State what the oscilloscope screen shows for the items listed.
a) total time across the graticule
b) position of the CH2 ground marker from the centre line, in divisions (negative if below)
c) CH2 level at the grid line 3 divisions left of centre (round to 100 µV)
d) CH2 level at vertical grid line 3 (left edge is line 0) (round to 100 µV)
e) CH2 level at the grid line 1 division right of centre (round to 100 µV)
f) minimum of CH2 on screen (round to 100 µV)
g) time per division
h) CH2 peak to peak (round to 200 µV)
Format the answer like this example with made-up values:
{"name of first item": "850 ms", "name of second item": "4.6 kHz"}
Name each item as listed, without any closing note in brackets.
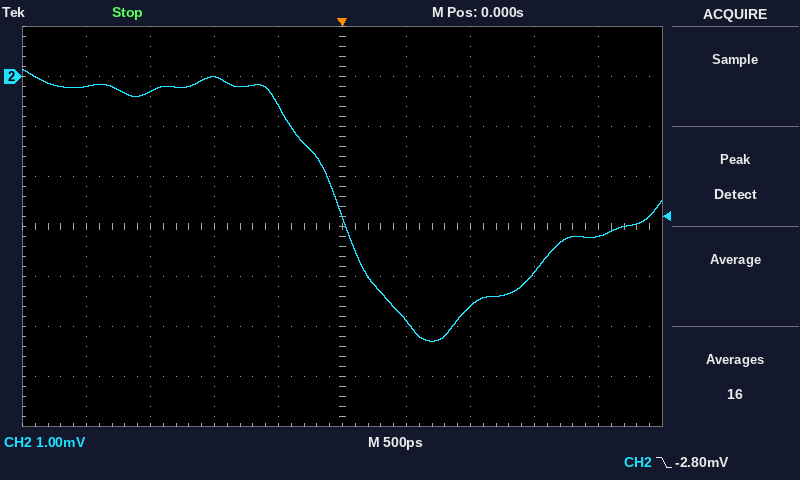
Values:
{"total time across the graticule": "5 ns", "position of the CH2 ground marker from the centre line, in divisions": "+3.0 div", "CH2 level at the grid line 3 divisions left of centre": "-300 µV", "CH2 level at vertical grid line 3 (left edge is line 0)": "0.0 mV", "CH2 level at the grid line 1 division right of centre": "-4.9 mV", "minimum of CH2 on screen": "-5.3 mV", "time per division": "500 ps", "CH2 peak to peak": "5.4 mV"}
